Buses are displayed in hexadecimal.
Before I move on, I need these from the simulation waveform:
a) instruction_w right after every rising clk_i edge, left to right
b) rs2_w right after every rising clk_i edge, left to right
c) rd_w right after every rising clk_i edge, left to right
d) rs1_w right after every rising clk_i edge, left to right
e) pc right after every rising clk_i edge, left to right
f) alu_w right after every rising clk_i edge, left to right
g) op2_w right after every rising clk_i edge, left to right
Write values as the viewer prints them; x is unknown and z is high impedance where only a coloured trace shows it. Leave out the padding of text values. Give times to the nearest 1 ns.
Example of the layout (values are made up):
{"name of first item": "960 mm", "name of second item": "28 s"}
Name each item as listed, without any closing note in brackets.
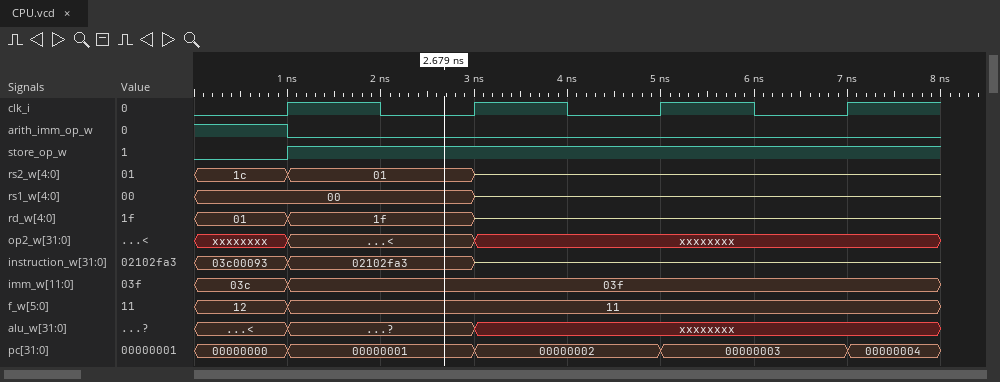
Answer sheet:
{"instruction_w right after every rising clk_i edge, left to right": "02102fa3, z, z, z", "rs2_w right after every rising clk_i edge, left to right": "01, z, z, z", "rd_w right after every rising clk_i edge, left to right": "1f, z, z, z", "rs1_w right after every rising clk_i edge, left to right": "00, z, z, z", "pc right after every rising clk_i edge, left to right": "00000001, 00000002, 00000003, 00000004", "alu_w right after every rising clk_i edge, left to right": "?, xxxxxxxx, xxxxxxxx, xxxxxxxx", "op2_w right after every rising clk_i edge, left to right": "<, xxxxxxxx, xxxxxxxx, xxxxxxxx"}
